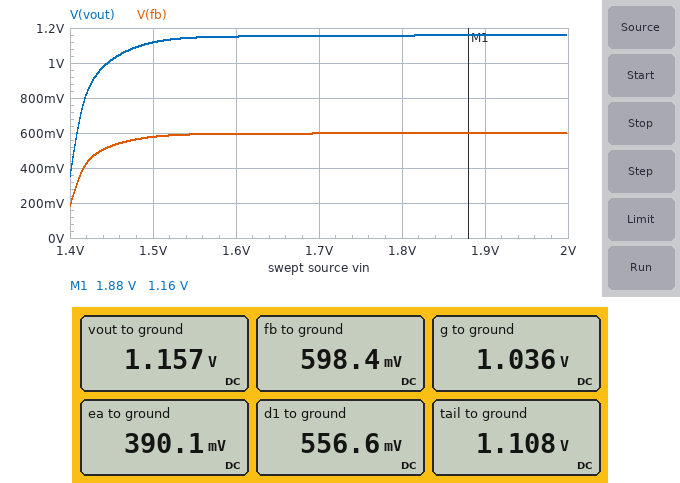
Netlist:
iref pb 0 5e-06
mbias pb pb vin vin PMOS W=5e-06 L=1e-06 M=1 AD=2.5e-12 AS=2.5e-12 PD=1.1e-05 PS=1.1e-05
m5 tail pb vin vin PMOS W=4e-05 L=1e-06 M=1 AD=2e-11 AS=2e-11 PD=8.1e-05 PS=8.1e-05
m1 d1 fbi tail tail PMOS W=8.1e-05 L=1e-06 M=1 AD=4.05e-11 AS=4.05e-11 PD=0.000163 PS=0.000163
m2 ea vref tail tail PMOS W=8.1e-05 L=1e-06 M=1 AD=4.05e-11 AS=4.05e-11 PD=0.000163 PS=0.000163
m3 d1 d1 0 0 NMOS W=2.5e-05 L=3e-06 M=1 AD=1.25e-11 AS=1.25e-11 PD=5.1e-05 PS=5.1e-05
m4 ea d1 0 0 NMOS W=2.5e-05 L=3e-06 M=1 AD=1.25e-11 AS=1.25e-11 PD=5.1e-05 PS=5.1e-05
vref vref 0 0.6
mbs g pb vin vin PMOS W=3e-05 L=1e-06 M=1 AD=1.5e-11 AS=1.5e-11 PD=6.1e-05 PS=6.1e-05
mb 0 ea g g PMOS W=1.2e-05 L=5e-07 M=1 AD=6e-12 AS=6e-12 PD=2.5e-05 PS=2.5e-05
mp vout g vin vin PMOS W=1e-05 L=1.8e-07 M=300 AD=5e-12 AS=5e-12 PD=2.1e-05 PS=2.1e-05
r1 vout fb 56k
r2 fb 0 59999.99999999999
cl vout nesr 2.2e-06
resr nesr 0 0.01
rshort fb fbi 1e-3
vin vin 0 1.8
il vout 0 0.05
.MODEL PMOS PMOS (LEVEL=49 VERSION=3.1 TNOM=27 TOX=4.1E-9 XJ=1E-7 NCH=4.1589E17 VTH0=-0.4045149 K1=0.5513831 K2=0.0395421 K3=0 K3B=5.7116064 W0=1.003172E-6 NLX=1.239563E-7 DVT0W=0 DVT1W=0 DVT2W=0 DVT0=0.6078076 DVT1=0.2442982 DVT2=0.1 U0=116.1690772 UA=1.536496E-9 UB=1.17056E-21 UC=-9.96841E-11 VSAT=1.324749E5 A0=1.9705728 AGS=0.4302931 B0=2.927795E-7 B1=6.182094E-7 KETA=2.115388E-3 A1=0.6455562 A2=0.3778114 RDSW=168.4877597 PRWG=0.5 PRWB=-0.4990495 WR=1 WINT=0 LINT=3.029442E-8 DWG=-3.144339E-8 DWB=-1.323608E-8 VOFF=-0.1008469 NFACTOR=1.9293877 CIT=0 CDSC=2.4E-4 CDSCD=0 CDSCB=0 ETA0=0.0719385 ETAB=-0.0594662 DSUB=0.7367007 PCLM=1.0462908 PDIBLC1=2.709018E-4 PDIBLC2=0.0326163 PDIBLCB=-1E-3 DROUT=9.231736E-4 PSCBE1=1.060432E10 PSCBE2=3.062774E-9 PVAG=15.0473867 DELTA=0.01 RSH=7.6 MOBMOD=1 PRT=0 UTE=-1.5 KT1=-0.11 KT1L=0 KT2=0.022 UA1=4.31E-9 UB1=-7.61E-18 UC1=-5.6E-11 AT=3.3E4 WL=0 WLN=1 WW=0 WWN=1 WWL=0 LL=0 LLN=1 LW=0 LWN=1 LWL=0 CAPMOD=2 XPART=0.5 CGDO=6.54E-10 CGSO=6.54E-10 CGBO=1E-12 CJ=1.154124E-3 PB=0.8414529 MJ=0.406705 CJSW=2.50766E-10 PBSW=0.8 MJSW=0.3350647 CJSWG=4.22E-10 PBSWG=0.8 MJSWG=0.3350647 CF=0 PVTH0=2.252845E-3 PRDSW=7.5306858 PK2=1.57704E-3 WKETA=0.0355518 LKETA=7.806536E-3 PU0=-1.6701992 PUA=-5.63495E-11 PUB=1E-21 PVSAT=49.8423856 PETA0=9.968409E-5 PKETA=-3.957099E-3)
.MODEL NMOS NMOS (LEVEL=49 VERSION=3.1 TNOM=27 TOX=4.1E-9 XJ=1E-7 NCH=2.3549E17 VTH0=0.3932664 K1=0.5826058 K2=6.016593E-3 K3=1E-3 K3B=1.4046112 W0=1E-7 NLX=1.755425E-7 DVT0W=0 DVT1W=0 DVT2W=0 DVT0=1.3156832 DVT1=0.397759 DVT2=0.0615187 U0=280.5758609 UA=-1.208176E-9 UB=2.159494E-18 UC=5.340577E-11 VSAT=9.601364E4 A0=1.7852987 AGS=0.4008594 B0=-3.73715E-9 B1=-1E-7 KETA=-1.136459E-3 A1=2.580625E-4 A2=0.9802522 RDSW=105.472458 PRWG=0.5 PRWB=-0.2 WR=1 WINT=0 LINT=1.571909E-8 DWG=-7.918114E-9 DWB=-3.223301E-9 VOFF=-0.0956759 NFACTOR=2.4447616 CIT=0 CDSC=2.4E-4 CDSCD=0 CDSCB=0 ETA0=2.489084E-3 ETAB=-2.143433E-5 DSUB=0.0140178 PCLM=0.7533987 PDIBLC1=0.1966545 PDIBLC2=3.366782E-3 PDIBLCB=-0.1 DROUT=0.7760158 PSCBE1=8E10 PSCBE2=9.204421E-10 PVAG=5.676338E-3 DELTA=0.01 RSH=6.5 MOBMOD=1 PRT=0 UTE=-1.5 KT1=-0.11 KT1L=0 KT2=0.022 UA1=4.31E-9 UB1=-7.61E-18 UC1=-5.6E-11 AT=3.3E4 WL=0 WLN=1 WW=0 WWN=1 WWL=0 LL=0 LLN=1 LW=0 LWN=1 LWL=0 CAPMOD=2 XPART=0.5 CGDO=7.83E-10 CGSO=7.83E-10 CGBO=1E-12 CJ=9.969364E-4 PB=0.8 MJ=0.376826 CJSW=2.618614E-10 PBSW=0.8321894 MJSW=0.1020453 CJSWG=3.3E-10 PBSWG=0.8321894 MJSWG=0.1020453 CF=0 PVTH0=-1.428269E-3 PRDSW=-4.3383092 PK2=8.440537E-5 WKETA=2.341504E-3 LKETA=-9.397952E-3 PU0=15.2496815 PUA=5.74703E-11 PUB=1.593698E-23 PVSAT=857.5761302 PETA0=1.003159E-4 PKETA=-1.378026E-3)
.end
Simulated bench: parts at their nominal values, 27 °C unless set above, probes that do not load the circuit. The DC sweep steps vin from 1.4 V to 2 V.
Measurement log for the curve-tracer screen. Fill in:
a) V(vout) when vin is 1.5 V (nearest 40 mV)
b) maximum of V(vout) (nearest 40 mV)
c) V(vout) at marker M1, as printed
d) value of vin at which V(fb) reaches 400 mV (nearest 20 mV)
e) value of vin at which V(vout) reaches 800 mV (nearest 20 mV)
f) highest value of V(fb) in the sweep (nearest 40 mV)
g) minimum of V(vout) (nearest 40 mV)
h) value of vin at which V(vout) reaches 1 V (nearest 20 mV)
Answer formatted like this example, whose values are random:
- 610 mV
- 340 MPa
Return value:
- 1.12 V
- 1.16 V
- 1.16 V
- 1.42 V
- 1.42 V
- 600 mV
- 360 mV
- 1.44 V
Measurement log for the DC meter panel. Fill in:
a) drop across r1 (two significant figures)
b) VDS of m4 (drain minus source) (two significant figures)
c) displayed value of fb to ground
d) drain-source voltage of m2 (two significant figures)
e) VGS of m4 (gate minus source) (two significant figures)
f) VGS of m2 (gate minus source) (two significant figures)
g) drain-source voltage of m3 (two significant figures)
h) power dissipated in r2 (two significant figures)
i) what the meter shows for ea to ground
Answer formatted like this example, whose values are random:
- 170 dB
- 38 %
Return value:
- 560 mV
- 390 mV
- 598.4 mV
- -720 mV
- 560 mV
- -510 mV
- 560 mV
- 6.0 µW
- 390.1 mV
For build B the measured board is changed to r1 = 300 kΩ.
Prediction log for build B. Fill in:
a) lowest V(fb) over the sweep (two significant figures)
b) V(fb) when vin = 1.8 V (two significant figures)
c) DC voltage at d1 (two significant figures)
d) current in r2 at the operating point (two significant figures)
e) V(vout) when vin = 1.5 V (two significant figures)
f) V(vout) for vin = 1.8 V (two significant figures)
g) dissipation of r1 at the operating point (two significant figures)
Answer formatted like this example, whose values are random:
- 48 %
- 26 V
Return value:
- 59 mV
- 290 mV
- 620 mV
- 4.8 µA
- 1.4 V
- 1.7 V
- 7.0 µW
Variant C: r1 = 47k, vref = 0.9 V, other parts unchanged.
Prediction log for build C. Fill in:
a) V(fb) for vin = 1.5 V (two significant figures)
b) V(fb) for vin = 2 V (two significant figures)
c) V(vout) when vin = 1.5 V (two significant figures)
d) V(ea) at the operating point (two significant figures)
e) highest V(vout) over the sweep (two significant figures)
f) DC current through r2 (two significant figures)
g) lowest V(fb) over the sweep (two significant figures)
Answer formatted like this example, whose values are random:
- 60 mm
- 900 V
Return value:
- 760 mV
- 900 mV
- 1.4 V
- 350 mV
- 1.6 V
- 15 µA
- 200 mV
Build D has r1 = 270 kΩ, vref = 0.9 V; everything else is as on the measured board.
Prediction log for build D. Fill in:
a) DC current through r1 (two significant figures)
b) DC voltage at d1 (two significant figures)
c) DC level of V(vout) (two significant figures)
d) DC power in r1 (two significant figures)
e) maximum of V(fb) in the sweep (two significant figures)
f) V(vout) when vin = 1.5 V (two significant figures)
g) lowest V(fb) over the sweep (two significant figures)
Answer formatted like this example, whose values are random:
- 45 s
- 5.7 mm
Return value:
- 5.3 µA
- 620 mV
- 1.7 V
- 7.5 µW
- 350 mV
- 1.4 V
- 64 mV
